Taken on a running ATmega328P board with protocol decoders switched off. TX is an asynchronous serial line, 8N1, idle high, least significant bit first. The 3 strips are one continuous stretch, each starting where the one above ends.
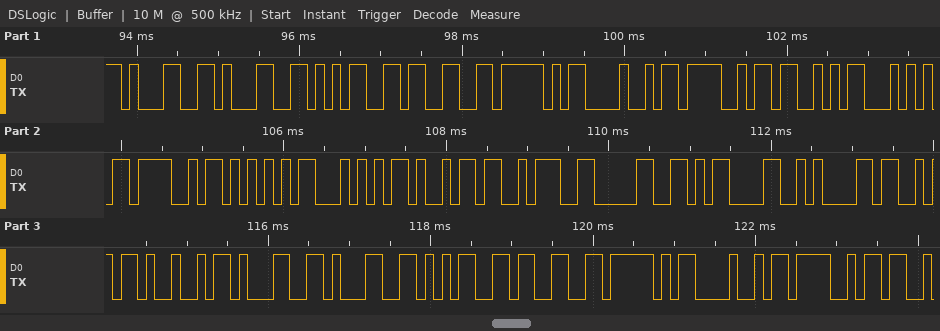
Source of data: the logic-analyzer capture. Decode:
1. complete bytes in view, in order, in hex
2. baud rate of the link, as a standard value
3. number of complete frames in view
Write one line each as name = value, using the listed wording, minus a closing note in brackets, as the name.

complete bytes in view, in order, in hex = 31 31 35 33 5F 48 4F 53 54 4F 55 54 69 3A 30 0D 0A 53 49 31 31 35 33 5F 48 4F
baud rate of the link, as a standard value = 9600 baud
number of complete frames in view = 26
